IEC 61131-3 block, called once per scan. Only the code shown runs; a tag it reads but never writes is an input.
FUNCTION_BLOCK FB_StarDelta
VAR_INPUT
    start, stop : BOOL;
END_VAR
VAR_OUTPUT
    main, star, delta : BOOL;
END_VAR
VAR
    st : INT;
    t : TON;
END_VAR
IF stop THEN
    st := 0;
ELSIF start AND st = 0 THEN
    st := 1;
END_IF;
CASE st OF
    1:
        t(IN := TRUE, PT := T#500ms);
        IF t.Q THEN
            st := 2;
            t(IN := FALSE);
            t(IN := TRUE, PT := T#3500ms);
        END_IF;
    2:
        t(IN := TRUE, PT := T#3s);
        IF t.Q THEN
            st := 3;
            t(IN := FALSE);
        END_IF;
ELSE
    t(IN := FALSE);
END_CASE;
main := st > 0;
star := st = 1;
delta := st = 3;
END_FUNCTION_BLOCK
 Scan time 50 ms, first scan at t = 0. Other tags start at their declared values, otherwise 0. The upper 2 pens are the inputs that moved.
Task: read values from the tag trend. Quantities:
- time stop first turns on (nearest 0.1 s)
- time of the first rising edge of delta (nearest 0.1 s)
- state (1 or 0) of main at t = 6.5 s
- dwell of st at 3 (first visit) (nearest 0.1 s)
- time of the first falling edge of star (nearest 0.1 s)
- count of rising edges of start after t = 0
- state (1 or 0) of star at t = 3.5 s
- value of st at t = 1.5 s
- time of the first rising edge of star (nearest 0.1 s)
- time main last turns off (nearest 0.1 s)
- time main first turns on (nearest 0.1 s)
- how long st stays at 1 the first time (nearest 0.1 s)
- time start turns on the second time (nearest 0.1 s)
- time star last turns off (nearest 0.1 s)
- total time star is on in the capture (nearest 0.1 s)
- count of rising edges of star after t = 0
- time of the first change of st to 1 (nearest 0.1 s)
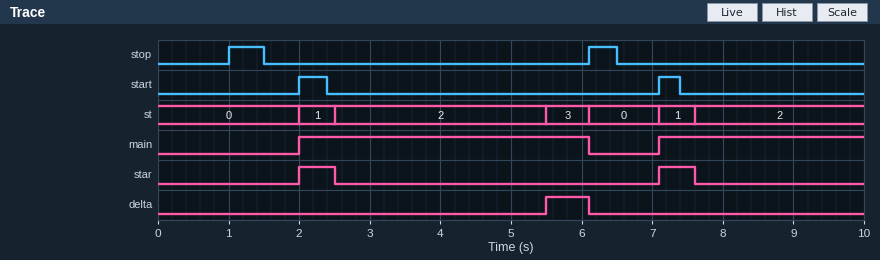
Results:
1.0 s
5.5 s
0
0.6 s
2.5 s
2
0
0
2.0 s
6.1 s
2.0 s
0.5 s
7.1 s
7.6 s
1.0 s
2
2.0 s
